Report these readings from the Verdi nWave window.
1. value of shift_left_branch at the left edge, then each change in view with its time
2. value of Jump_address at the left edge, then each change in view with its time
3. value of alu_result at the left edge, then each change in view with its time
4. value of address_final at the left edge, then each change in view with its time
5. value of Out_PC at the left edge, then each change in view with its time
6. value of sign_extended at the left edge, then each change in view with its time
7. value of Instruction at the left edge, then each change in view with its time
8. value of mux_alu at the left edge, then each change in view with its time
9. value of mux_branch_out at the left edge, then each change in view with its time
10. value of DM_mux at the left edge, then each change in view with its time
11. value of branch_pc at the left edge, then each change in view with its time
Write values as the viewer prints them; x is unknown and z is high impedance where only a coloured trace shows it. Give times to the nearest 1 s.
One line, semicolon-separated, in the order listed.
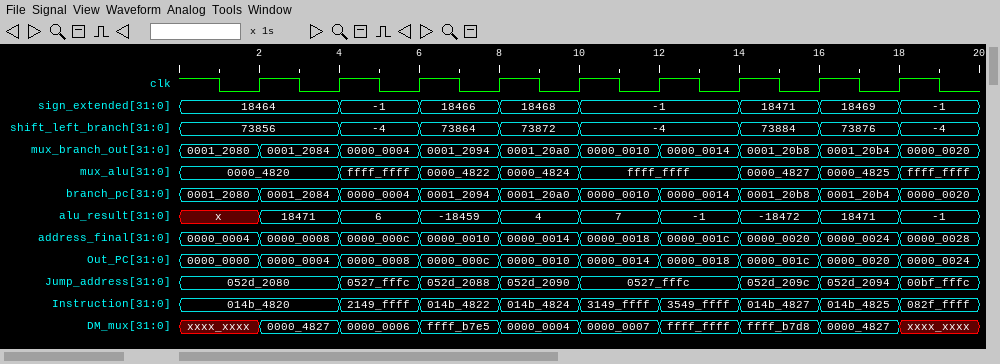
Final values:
73856, -4 at 4 s, 73864 at 6 s, 73872 at 8 s, -4 at 10 s, 73884 at 14 s, 73876 at 16 s, -4 at 18 s; 052d_2080, 0527_fffc at 4 s, 052d_2088 at 6 s, 052d_2090 at 8 s, 0527_fffc at 10 s, 052d_209c at 14 s, 052d_2094 at 16 s, 00bf_fffc at 18 s; x, 18471 at 2 s, 6 at 4 s, -18459 at 6 s, 4 at 8 s, 7 at 10 s, -1 at 12 s, -18472 at 14 s, 18471 at 16 s, -1 at 18 s; 0000_0004, 0000_0008 at 2 s, 0000_000c at 4 s, 0000_0010 at 6 s, 0000_0014 at 8 s, 0000_0018 at 10 s, 0000_001c at 12 s, 0000_0020 at 14 s, 0000_0024 at 16 s, 0000_0028 at 18 s; 0000_0000, 0000_0004 at 2 s, 0000_0008 at 4 s, 0000_000c at 6 s, 0000_0010 at 8 s, 0000_0014 at 10 s, 0000_0018 at 12 s, 0000_001c at 14 s, 0000_0020 at 16 s, 0000_0024 at 18 s; 18464, -1 at 4 s, 18466 at 6 s, 18468 at 8 s, -1 at 10 s, 18471 at 14 s, 18469 at 16 s, -1 at 18 s; 014b_4820, 2149_ffff at 4 s, 014b_4822 at 6 s, 014b_4824 at 8 s, 3149_ffff at 10 s, 3549_ffff at 12 s, 014b_4827 at 14 s, 014b_4825 at 16 s, 082f_ffff at 18 s; 0000_4820, ffff_ffff at 4 s, 0000_4822 at 6 s, 0000_4824 at 8 s, ffff_ffff at 10 s, 0000_4827 at 14 s, 0000_4825 at 16 s, ffff_ffff at 18 s; 0001_2080, 0001_2084 at 2 s, 0000_0004 at 4 s, 0001_2094 at 6 s, 0001_20a0 at 8 s, 0000_0010 at 10 s, 0000_0014 at 12 s, 0001_20b8 at 14 s, 0001_20b4 at 16 s, 0000_0020 at 18 s; xxxx_xxxx, 0000_4827 at 2 s, 0000_0006 at 4 s, ffff_b7e5 at 6 s, 0000_0004 at 8 s, 0000_0007 at 10 s, ffff_ffff at 12 s, ffff_b7d8 at 14 s, 0000_4827 at 16 s, xxxx_xxxx at 18 s; 0001_2080, 0001_2084 at 2 s, 0000_0004 at 4 s, 0001_2094 at 6 s, 0001_20a0 at 8 s, 0000_0010 at 10 s, 0000_0014 at 12 s, 0001_20b8 at 14 s, 0001_20b4 at 16 s, 0000_0020 at 18 s
